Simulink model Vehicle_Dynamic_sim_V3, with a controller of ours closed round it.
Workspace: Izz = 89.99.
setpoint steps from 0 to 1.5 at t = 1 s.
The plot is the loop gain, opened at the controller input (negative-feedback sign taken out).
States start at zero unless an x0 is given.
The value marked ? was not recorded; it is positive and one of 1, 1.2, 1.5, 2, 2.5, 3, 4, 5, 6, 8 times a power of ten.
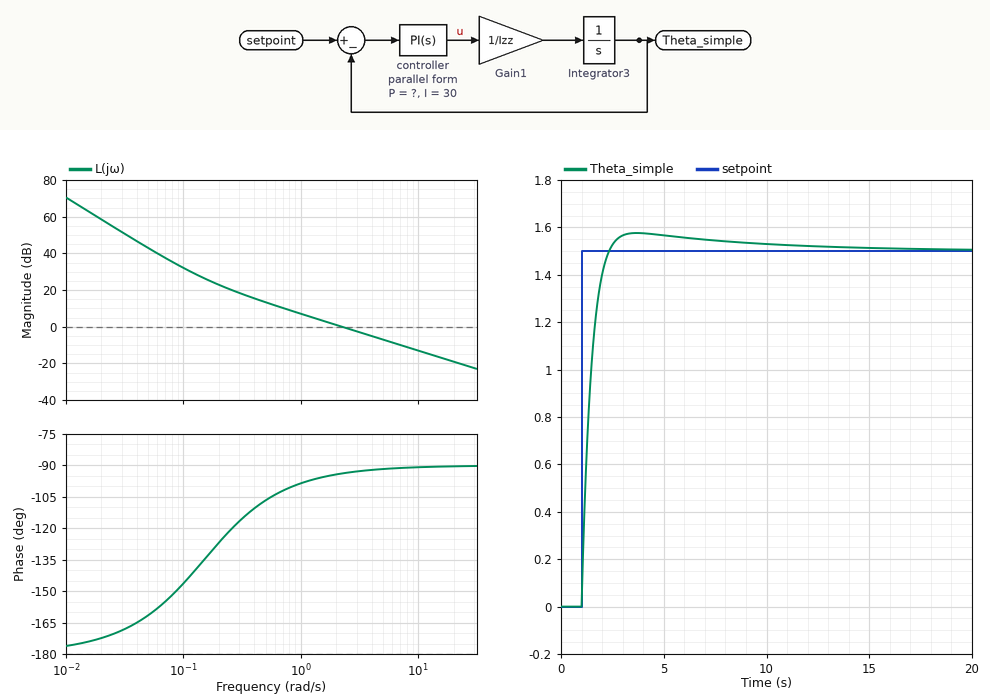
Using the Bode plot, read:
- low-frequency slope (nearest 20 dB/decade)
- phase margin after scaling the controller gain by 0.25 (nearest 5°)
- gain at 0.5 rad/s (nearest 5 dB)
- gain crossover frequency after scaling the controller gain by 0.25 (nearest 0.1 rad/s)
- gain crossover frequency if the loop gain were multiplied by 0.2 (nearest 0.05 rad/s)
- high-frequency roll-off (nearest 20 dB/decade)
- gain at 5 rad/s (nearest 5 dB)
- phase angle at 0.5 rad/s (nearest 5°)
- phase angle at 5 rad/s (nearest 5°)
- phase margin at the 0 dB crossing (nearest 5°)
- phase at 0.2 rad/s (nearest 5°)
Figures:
-40 dB/decade
75°
15 dB
0.6 rad/s
0.45 rad/s
-20 dB/decade
-5 dB
-105°
-90°
85°
-125°
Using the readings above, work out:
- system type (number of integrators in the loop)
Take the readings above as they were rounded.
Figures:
2
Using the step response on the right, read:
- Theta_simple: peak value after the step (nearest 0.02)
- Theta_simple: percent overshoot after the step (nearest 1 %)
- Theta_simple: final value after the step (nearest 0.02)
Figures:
1.58
5 %
1.50
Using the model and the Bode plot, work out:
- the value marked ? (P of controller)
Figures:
200
